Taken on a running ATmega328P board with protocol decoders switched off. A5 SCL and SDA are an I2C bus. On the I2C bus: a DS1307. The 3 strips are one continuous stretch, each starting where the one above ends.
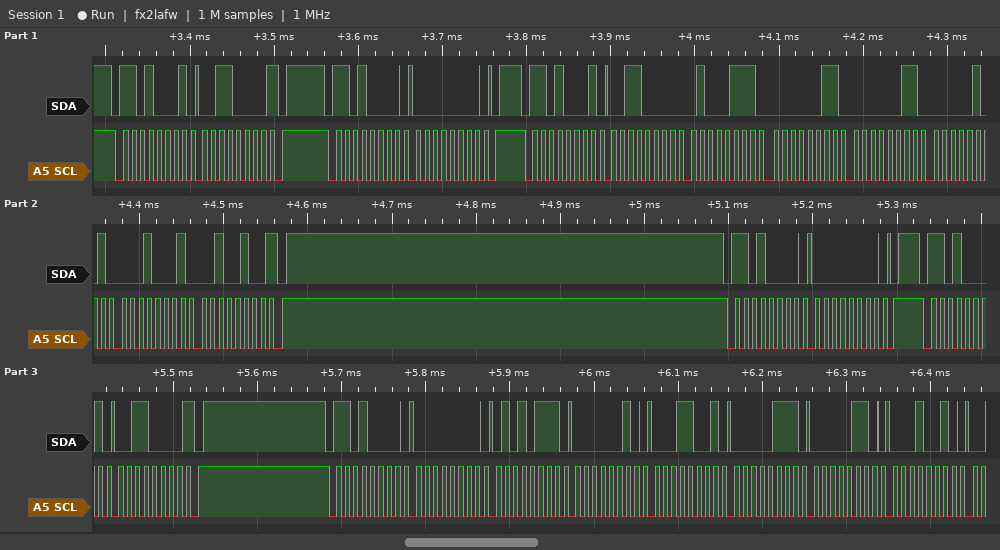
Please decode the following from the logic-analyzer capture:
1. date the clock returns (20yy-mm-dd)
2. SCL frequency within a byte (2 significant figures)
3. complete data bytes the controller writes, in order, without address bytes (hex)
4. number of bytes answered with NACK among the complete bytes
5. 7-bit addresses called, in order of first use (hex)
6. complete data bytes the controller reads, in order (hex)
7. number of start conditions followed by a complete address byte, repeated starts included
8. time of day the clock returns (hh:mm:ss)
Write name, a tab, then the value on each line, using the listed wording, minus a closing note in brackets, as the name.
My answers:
date the clock returns	2024-11-05
SCL frequency within a byte	100 kHz
complete data bytes the controller writes, in order, without address bytes	00 00 00 57 02 19 07 06 12
number of bytes answered with NACK among the complete bytes	3
7-bit addresses called, in order of first use	0x68
complete data bytes the controller reads, in order	30 30 47 03 03 05 11 24 30
number of start conditions followed by a complete address byte, repeated starts included	6
time of day the clock returns	03:47:30
